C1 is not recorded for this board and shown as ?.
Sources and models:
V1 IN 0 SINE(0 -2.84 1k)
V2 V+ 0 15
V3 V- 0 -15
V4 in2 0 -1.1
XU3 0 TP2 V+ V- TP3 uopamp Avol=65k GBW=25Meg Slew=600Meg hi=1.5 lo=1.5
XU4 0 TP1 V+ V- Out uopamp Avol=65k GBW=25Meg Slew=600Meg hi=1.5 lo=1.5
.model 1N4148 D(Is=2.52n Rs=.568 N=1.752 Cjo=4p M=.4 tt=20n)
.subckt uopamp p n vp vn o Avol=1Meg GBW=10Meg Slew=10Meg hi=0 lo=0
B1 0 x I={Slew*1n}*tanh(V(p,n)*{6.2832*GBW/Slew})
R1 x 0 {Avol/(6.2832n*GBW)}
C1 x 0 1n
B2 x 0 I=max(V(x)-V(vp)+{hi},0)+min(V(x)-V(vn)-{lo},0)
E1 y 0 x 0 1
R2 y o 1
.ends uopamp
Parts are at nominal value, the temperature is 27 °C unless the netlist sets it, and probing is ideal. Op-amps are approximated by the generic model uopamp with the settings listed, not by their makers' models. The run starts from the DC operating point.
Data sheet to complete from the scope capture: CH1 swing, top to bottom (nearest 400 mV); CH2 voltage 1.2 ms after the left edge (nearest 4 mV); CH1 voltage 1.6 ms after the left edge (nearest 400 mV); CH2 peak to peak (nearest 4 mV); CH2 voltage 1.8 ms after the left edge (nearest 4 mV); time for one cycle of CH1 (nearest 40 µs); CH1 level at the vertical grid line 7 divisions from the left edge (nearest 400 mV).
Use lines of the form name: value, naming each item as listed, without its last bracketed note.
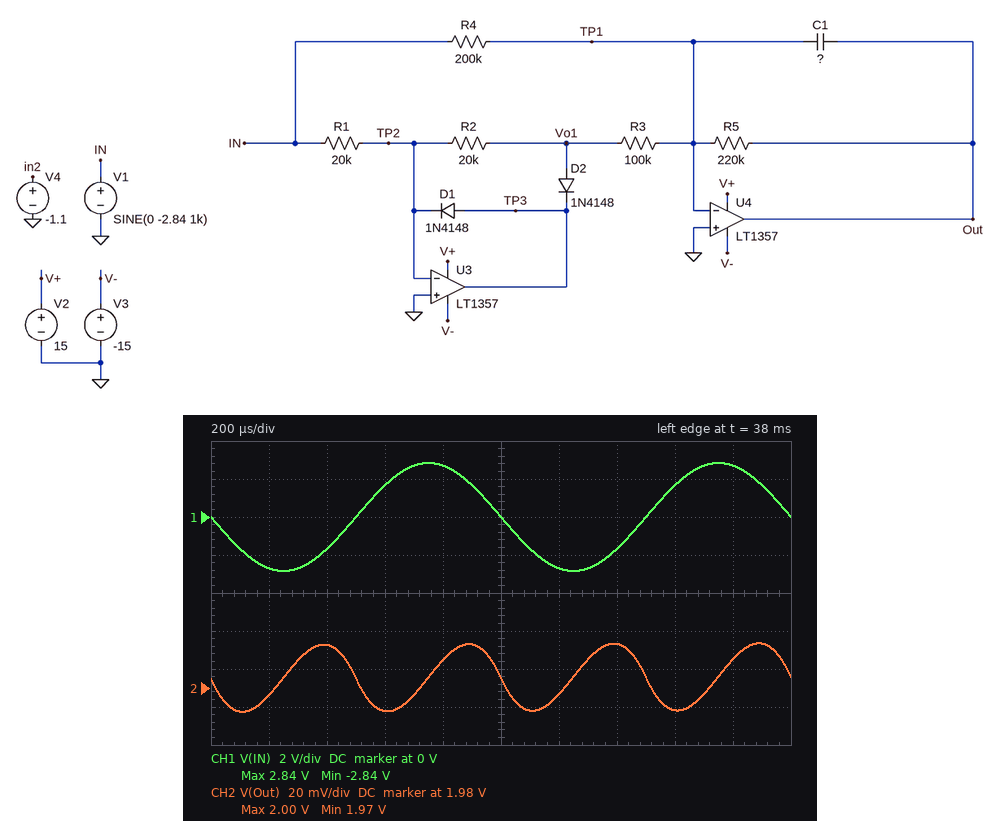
CH1 swing, top to bottom: 5.6 V
CH2 voltage 1.2 ms after the left edge: 1.976 V
CH1 voltage 1.6 ms after the left edge: 1.6 V
CH2 peak to peak: 36 mV
CH2 voltage 1.8 ms after the left edge: 1.996 V
time for one cycle of CH1: 1.00 ms
CH1 level at the vertical grid line 7 divisions from the left edge: -1.6 V
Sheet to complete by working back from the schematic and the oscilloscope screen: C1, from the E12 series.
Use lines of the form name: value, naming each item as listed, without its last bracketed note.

C1, from the E12 series: 27 nF
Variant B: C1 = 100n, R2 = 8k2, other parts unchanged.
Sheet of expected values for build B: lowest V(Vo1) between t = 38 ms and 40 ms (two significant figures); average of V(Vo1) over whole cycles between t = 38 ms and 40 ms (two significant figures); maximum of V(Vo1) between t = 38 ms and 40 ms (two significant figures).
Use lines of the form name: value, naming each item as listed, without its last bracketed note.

lowest V(Vo1) between t = 38 ms and 40 ms: -1.2 V
average of V(Vo1) over whole cycles between t = 38 ms and 40 ms: -370 mV
maximum of V(Vo1) between t = 38 ms and 40 ms: 6.2 mV
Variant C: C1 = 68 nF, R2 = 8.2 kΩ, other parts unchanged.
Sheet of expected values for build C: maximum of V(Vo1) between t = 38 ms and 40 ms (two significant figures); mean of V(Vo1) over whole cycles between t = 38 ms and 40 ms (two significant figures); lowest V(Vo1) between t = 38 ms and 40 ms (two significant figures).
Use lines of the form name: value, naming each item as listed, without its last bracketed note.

maximum of V(Vo1) between t = 38 ms and 40 ms: 6.2 mV
mean of V(Vo1) over whole cycles between t = 38 ms and 40 ms: -370 mV
lowest V(Vo1) between t = 38 ms and 40 ms: -1.2 V
